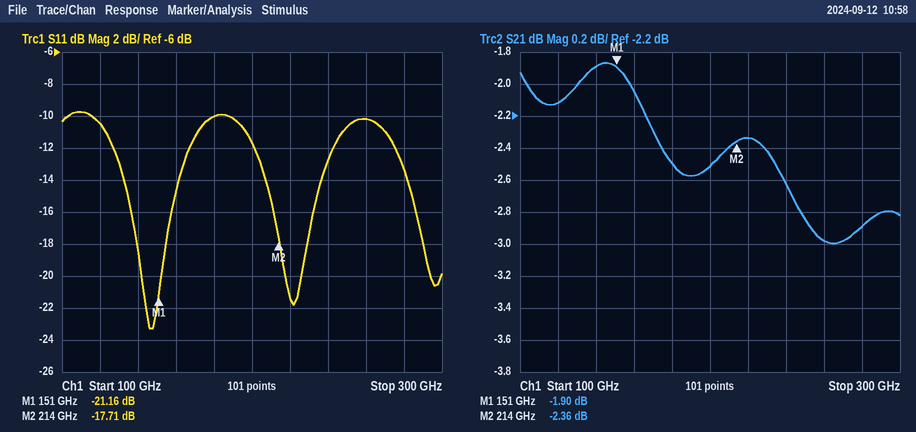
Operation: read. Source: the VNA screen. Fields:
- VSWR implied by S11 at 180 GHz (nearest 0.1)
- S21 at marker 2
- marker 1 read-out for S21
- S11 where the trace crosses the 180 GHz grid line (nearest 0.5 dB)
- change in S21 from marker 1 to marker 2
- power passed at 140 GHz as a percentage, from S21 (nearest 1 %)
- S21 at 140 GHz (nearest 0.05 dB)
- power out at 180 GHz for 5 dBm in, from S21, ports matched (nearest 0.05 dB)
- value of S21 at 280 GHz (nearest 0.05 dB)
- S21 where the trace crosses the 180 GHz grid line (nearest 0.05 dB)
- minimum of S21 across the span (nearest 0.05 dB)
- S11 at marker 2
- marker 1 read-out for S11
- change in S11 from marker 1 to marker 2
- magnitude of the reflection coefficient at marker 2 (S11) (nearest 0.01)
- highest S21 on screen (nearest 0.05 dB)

1.9
-2.36 dB
-1.90 dB
-10.0 dB
-0.46 dB
65 %
-1.90 dB
2.50 dBm
-2.90 dB
-2.50 dB
-3.00 dB
-17.71 dB
-21.16 dB
3.45 dB
0.13
-1.85 dB
